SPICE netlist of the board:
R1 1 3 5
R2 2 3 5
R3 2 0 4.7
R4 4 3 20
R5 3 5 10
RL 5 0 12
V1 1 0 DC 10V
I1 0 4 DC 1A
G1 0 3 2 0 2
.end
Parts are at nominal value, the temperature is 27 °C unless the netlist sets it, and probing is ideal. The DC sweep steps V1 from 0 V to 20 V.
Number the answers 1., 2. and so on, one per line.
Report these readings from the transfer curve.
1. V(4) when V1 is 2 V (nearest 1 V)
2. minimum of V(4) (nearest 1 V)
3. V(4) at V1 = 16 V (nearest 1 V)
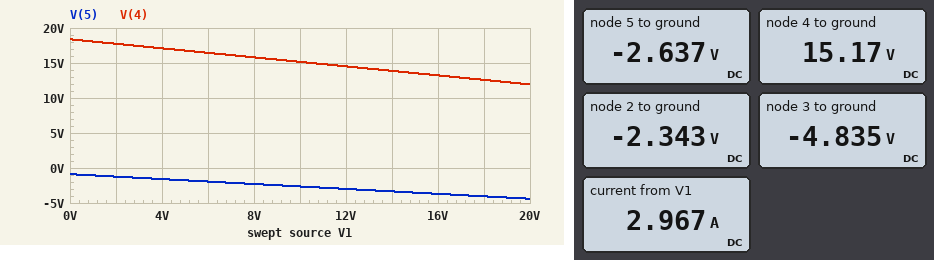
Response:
1. 18 V
2. 12 V
3. 13 V
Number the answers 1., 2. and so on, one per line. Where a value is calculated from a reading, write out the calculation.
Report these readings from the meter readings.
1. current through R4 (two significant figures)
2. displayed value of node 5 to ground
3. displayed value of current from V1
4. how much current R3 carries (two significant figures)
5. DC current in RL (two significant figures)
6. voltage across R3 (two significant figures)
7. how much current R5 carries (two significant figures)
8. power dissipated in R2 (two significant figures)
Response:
1. (15.17 V - (-4.835 V)) / 20 Ω = 1.0 A
2. -2.637 V
3. 2.967 A
4. (0 V - (-2.343 V)) / 4.7 Ω = 500 mA
5. (0 V - (-2.637 V)) / 12 Ω = 220 mA
6. 0 V - (-2.343 V) = 2.3 V
7. (-2.637 V - (-4.835 V)) / 10 Ω = 220 mA
8. (-2.343 V - (-4.835 V))^2 / 5 Ω = 1.2 W
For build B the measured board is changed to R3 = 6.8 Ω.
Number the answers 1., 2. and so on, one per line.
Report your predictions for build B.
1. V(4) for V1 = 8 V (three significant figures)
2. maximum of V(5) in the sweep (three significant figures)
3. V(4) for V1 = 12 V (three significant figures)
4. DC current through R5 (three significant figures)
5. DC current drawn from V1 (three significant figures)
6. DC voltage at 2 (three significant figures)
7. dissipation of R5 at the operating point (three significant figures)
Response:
1. 16.8 V
2. -663 mV
3. 15.9 V
4. 166 mA
5. 2.73 A
6. -2.10 V
7. 275 mW
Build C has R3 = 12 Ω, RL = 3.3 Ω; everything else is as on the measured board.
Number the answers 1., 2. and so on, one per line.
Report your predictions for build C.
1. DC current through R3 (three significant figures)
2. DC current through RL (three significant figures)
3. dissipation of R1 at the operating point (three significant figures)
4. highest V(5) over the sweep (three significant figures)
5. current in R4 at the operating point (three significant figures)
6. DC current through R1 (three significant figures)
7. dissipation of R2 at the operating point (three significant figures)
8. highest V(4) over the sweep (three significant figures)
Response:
1. 164 mA
2. 209 mA
3. 32.7 W
4. -230 mV
5. 1.00 A
6. 2.56 A
7. 134 mW
8. 19.1 V
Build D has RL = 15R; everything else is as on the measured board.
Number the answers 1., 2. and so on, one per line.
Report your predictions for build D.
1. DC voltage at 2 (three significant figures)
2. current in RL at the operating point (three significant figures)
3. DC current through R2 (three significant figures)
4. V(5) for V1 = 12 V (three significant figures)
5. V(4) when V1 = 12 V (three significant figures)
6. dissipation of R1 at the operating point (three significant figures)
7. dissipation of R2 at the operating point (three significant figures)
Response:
1. -2.32 V
2. 192 mA
3. 494 mA
4. -3.26 V
5. 14.6 V
6. 43.8 W
7. 1.22 W
